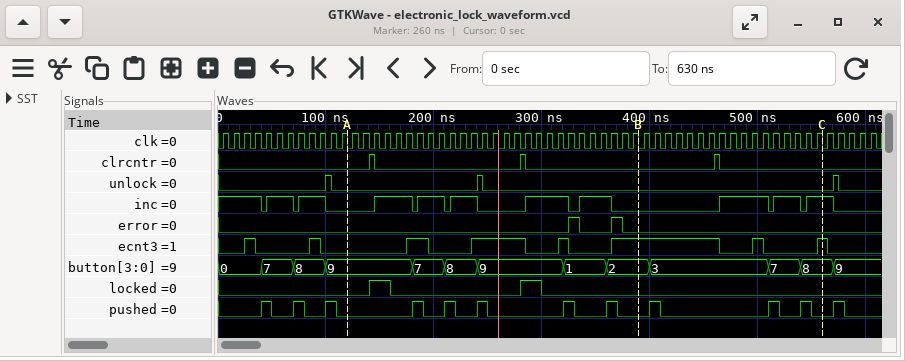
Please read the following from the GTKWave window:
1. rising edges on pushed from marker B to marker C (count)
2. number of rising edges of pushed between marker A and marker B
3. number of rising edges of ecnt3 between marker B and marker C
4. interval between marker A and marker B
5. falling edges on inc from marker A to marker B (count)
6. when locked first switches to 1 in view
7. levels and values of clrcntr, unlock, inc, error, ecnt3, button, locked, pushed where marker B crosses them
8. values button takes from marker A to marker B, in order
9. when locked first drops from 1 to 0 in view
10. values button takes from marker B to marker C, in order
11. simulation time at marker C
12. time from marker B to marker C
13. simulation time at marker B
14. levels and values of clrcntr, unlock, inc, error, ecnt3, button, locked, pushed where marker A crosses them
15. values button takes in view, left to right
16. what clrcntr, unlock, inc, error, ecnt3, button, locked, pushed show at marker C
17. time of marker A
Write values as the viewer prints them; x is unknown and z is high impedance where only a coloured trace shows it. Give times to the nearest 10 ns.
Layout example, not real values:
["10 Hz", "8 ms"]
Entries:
["3", "5", "2", "270 ns", "5", "140 ns", "clrcntr=0, unlock=0, inc=0, error=0, ecnt3=1, button=2, locked=0, pushed=0", "9, 7, 8, 9, 1, 2", "160 ns", "2, 3, 7, 8", "560 ns", "170 ns", "390 ns", "clrcntr=0, unlock=0, inc=0, error=0, ecnt3=0, button=9, locked=0, pushed=0", "0, 7, 8, 9, 7, 8, 9, 1, 2, 3, 7, 8, 9", "clrcntr=0, unlock=0, inc=1, error=0, ecnt3=1, button=8, locked=0, pushed=0", "120 ns"]
